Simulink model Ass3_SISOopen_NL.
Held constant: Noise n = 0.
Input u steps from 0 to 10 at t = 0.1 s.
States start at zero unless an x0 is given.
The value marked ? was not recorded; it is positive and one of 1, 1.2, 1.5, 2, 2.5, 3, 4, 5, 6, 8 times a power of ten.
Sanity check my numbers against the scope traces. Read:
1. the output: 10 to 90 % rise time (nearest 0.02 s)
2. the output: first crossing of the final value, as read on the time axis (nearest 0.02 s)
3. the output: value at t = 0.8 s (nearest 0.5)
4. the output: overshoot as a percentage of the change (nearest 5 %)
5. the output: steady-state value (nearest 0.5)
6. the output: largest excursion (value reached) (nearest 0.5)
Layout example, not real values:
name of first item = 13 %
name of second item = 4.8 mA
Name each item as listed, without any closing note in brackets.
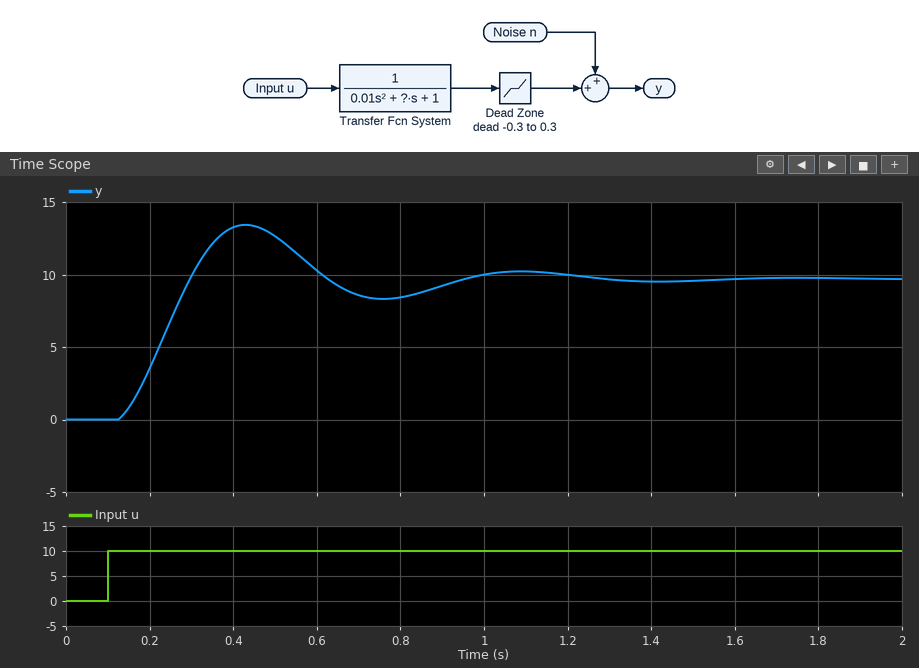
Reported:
the output: 10 to 90 % rise time = 0.12 s
the output: first crossing of the final value, as read on the time axis = 0.30 s
the output: value at t = 0.8 s = 8.5
the output: overshoot as a percentage of the change = 40 %
the output: steady-state value = 9.5
the output: largest excursion (value reached) = 13.5
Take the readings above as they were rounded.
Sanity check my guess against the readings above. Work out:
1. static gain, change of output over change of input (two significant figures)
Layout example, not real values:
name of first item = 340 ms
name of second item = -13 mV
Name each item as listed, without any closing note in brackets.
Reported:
static gain, change of output over change of input = 0.95
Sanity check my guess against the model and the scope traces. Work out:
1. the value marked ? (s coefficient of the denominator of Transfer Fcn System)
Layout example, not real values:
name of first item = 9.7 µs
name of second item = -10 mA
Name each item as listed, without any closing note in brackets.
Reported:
the value marked ? = 0.06
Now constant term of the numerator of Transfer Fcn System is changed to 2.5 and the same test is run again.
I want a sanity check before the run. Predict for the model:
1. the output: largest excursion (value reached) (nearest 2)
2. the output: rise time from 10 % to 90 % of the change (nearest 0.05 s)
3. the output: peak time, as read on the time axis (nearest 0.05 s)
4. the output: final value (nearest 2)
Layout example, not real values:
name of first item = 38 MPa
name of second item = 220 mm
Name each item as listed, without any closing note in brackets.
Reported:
the output: largest excursion (value reached) = 34
the output: rise time from 10 % to 90 % of the change = 0.15 s
the output: peak time, as read on the time axis = 0.45 s
the output: final value = 24
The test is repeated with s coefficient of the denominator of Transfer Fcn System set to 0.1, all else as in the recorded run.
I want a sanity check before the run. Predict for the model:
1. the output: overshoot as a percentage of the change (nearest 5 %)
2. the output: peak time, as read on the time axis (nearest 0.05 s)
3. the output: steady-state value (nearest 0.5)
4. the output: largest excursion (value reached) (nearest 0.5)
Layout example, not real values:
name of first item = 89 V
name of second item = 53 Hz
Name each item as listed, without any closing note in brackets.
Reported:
the output: overshoot as a percentage of the change = 15 %
the output: peak time, as read on the time axis = 0.45 s
the output: steady-state value = 9.5
the output: largest excursion (value reached) = 11.5
